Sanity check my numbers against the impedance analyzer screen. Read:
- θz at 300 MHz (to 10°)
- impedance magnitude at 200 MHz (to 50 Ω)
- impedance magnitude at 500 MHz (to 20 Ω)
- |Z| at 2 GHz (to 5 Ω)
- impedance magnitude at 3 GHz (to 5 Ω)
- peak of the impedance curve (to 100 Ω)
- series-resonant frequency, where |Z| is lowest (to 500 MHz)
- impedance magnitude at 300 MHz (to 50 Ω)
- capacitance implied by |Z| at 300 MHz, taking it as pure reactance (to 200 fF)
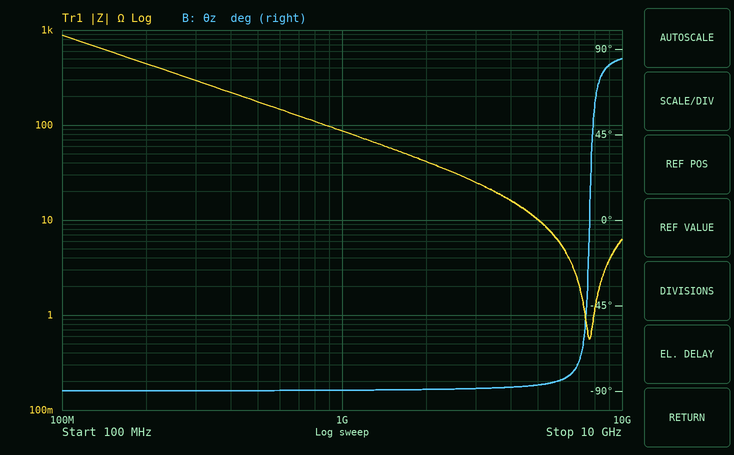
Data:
-90°
450 Ω
180 Ω
40 Ω
25 Ω
900 Ω
7.5 GHz
300 Ω
1.8 pF
